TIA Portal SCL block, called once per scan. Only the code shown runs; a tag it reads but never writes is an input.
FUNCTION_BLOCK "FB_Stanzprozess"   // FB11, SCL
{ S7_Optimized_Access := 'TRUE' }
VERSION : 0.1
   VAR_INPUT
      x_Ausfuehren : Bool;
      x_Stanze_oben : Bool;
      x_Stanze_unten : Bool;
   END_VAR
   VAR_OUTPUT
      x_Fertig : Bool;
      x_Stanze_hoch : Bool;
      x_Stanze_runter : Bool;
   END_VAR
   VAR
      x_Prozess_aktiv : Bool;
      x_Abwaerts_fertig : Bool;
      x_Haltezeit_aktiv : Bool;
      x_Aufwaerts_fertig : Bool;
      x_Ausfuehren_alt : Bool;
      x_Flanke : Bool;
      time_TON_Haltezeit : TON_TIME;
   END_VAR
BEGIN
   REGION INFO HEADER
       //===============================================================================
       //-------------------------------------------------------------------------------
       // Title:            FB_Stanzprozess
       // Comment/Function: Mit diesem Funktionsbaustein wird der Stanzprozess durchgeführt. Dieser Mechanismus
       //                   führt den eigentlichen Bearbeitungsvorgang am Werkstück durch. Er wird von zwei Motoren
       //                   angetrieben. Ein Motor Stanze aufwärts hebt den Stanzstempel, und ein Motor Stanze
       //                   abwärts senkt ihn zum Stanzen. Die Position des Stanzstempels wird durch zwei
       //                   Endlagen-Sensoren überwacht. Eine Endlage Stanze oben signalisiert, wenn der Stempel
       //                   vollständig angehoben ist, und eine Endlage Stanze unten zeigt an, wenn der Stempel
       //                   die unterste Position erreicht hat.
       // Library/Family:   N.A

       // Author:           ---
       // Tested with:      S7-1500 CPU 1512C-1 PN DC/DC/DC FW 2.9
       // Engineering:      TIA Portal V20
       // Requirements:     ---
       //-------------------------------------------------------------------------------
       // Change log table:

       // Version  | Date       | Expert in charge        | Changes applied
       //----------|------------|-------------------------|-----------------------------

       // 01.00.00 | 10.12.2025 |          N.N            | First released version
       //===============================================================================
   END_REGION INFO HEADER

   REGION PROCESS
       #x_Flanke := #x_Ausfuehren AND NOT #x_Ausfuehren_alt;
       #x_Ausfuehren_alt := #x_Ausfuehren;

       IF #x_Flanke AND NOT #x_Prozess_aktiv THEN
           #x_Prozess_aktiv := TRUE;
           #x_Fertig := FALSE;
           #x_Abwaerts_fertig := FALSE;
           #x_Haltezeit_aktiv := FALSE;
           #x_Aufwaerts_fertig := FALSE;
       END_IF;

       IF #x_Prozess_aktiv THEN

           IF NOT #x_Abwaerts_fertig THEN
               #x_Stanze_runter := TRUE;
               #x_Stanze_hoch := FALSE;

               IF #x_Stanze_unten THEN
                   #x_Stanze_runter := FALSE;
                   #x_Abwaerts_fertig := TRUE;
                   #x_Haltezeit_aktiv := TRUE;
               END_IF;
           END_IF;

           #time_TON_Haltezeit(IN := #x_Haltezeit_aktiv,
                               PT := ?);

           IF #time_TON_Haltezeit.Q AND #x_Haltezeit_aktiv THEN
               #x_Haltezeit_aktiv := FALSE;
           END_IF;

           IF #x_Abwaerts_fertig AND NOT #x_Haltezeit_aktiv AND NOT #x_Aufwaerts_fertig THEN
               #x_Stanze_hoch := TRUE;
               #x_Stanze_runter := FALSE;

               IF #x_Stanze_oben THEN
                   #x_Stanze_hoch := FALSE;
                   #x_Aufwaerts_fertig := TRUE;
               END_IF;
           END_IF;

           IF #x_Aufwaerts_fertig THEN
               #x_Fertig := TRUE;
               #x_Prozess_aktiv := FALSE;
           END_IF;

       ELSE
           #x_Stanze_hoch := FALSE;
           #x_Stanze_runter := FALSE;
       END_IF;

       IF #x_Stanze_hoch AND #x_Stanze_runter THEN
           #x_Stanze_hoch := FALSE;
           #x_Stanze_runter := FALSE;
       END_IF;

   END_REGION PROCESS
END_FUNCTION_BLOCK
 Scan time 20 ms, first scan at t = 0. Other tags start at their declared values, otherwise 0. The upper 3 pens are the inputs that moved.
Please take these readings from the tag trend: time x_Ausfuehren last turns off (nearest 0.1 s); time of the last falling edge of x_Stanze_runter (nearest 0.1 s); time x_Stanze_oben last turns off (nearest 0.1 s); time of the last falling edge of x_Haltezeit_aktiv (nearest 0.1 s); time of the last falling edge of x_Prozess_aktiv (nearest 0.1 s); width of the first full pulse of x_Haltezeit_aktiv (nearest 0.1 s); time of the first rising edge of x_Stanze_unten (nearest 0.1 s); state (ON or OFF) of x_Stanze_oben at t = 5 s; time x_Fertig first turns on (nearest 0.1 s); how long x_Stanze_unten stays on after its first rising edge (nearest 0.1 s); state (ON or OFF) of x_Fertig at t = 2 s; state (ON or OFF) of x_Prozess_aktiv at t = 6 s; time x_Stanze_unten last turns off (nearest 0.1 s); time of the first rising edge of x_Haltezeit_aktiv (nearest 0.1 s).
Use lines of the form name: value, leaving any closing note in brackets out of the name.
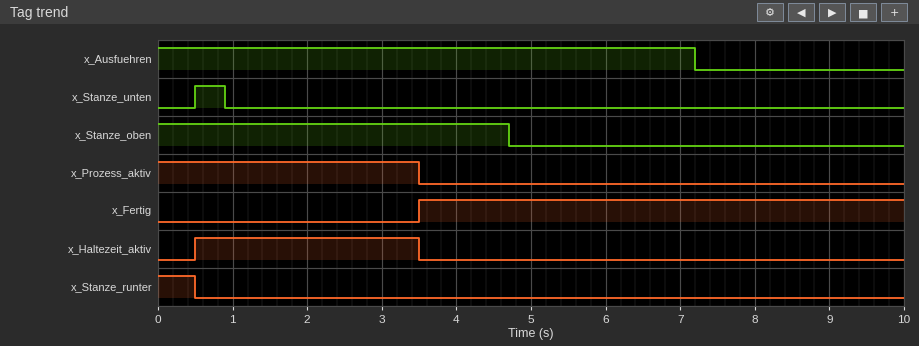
time x_Ausfuehren last turns off: 7.2 s
time of the last falling edge of x_Stanze_runter: 0.5 s
time x_Stanze_oben last turns off: 4.7 s
time of the last falling edge of x_Haltezeit_aktiv: 3.5 s
time of the last falling edge of x_Prozess_aktiv: 3.5 s
width of the first full pulse of x_Haltezeit_aktiv: 3.0 s
time of the first rising edge of x_Stanze_unten: 0.5 s
state (ON or OFF) of x_Stanze_oben at t = 5 s: OFF
time x_Fertig first turns on: 3.5 s
how long x_Stanze_unten stays on after its first rising edge: 0.4 s
state (ON or OFF) of x_Fertig at t = 2 s: OFF
state (ON or OFF) of x_Prozess_aktiv at t = 6 s: OFF
time x_Stanze_unten last turns off: 0.9 s
time of the first rising edge of x_Haltezeit_aktiv: 0.5 s
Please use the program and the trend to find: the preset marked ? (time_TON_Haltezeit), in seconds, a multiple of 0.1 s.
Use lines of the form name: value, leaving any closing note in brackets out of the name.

the preset marked ? (time_TON_Haltezeit), in seconds, a multiple of 0.1 s: 3.0 s
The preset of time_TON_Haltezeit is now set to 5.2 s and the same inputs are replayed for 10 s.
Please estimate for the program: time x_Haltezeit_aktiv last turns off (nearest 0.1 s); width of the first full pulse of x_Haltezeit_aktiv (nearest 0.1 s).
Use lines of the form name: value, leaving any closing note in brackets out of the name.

time x_Haltezeit_aktiv last turns off: 5.7 s
width of the first full pulse of x_Haltezeit_aktiv: 5.2 s
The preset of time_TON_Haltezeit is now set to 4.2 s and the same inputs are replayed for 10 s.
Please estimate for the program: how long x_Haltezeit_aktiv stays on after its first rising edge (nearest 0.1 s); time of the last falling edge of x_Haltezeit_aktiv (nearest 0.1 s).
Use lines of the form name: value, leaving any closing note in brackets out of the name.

how long x_Haltezeit_aktiv stays on after its first rising edge: 4.2 s
time of the last falling edge of x_Haltezeit_aktiv: 4.7 s
